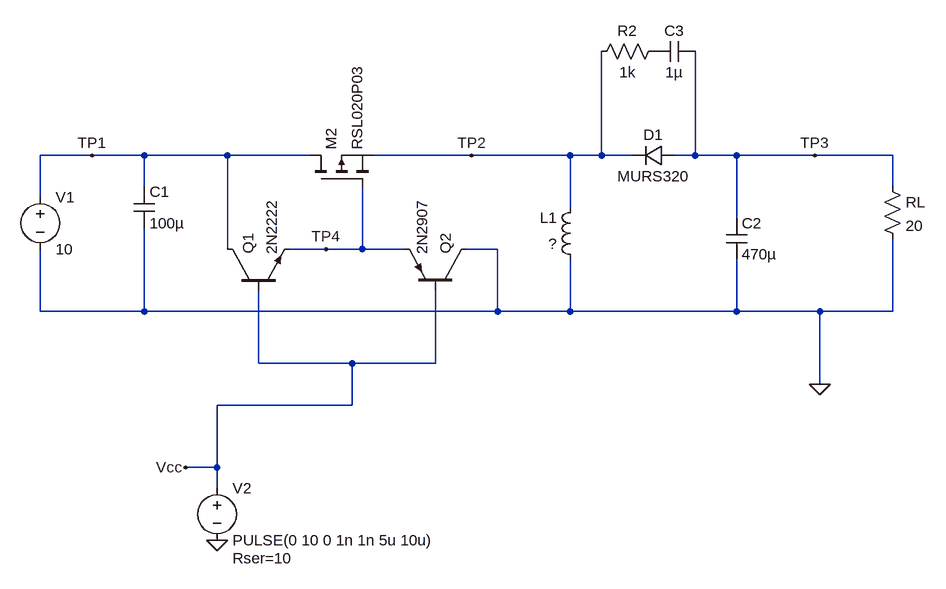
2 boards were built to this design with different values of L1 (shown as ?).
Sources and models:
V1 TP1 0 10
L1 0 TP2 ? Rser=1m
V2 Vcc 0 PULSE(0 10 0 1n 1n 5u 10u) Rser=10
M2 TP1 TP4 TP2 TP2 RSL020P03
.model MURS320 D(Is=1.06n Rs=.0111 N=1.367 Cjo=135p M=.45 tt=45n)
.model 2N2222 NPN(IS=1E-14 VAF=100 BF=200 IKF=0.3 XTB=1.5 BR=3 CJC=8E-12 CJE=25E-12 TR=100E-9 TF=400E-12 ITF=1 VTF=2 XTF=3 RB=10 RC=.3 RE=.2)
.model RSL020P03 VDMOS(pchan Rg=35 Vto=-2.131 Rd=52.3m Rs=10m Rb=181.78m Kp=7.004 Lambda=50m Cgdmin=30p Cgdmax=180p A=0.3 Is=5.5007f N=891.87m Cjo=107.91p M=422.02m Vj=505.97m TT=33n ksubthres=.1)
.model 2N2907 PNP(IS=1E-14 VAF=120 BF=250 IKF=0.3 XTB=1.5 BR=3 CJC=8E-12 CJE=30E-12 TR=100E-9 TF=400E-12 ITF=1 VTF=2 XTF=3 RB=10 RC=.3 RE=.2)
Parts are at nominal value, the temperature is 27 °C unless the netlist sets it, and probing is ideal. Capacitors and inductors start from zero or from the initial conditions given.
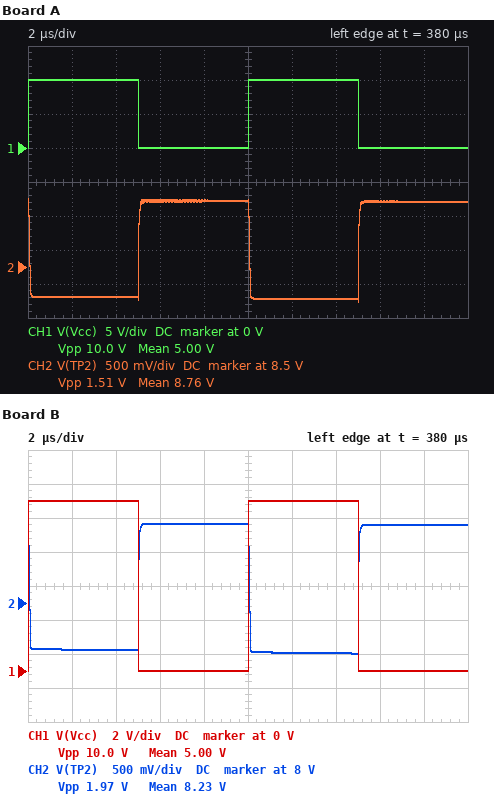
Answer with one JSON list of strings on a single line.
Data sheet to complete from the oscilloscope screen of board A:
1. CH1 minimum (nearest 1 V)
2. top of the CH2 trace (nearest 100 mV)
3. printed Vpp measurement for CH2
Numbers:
["0 V", "9.5 V", "1.51 V"]
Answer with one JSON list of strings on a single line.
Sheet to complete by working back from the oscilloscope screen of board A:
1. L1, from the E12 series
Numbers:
["560 µH"]
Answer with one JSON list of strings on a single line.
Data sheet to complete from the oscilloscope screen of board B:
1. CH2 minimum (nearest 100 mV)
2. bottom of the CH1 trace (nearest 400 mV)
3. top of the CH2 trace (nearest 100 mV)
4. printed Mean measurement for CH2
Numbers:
["7.2 V", "0 V", "9.2 V", "8.23 V"]
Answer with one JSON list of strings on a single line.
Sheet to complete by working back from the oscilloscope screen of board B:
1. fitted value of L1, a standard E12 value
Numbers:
["330 µH"]
